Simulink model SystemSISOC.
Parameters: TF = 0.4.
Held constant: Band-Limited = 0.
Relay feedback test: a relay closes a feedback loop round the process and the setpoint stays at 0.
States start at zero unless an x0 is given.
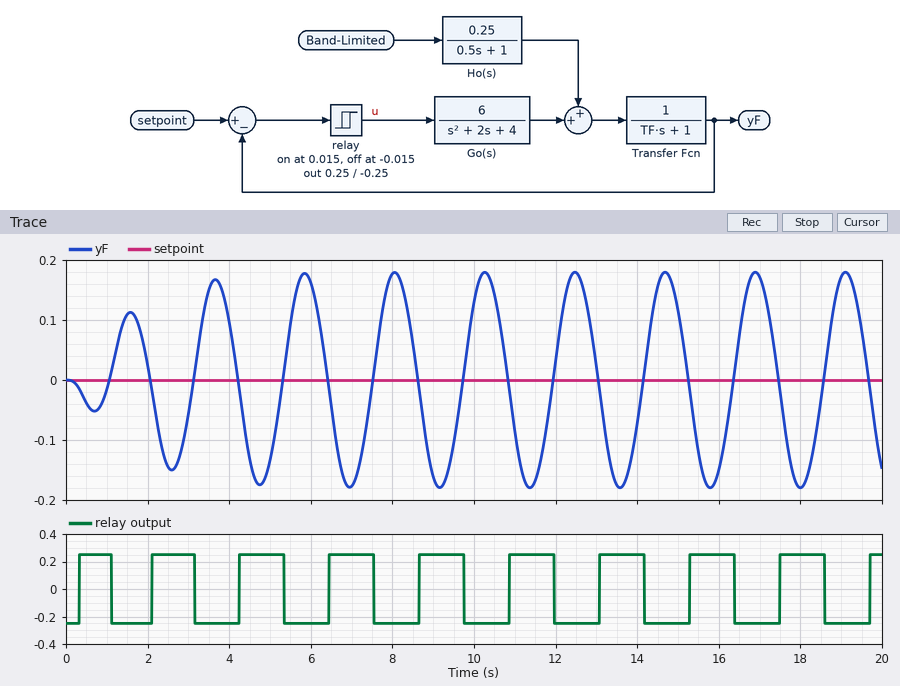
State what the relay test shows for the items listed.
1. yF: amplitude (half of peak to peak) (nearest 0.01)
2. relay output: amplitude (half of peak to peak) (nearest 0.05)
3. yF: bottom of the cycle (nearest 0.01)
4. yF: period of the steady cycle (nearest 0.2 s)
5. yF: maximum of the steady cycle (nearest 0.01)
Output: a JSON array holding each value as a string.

["0.18", "0.25", "-0.18", "2.2 s", "0.18"]
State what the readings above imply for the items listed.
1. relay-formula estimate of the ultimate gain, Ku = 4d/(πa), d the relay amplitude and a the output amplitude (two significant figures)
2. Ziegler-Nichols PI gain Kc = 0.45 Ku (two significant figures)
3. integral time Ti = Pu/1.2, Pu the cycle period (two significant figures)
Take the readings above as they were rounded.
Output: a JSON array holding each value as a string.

["1.8", "0.81", "1.8 s"]
